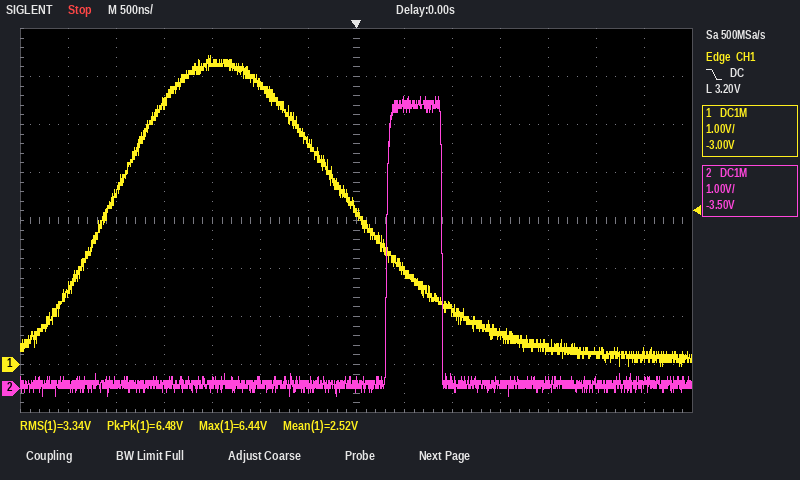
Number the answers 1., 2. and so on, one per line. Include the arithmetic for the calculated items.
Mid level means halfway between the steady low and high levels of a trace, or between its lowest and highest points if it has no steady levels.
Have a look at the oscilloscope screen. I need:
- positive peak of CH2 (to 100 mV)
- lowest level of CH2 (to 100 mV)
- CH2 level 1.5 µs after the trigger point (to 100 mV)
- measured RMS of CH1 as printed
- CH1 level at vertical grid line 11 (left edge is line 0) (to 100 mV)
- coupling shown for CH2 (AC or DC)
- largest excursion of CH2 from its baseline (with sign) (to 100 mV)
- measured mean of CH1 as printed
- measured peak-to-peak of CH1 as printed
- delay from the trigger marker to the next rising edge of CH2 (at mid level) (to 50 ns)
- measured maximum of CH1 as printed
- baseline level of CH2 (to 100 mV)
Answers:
1. 6.1 V
2. -200 mV
3. 100 mV
4. 3.34 V
5. 400 mV
6. DC
7. 6.1 V − (100 mV) = +6.0 V
8. 2.52 V
9. 6.48 V
10. 300 ns
11. 6.44 V
12. 100 mV
